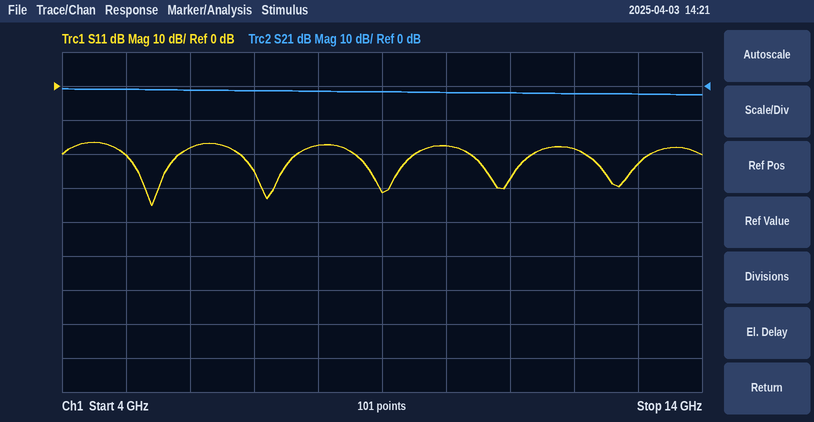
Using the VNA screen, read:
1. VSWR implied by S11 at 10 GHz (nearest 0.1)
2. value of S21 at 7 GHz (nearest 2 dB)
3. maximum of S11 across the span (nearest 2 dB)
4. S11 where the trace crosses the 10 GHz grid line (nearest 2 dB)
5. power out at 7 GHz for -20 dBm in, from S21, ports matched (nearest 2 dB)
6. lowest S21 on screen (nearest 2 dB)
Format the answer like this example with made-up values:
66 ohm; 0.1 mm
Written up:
1.3; -2 dB; -16 dB; -18 dB; -22 dBm; -2 dB
